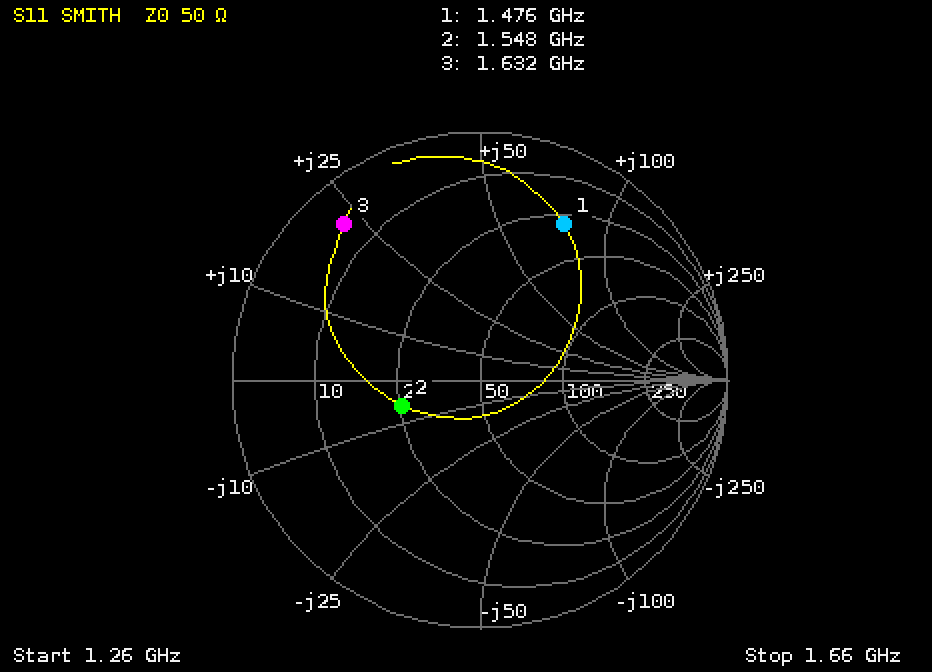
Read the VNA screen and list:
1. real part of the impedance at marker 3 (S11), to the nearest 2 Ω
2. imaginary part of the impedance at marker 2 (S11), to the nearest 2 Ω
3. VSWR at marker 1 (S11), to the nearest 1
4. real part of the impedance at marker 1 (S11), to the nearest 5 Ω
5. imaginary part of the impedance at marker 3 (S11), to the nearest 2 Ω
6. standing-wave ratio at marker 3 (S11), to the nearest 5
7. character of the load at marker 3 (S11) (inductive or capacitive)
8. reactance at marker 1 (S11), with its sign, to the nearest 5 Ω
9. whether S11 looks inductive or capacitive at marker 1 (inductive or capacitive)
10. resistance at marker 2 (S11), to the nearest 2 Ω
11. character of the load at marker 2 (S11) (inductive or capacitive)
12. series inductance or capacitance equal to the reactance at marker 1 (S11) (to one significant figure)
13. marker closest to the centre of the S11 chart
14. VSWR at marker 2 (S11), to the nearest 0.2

6 Ω
-6 Ω
6
30 Ω
+22 Ω
10
inductive
+75 Ω
inductive
26 Ω
capacitive
8 nH
marker 2
2.0
